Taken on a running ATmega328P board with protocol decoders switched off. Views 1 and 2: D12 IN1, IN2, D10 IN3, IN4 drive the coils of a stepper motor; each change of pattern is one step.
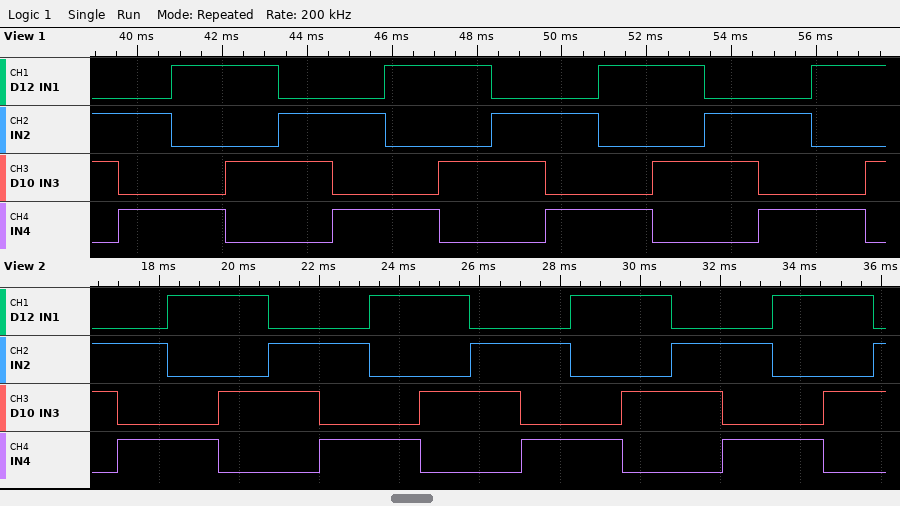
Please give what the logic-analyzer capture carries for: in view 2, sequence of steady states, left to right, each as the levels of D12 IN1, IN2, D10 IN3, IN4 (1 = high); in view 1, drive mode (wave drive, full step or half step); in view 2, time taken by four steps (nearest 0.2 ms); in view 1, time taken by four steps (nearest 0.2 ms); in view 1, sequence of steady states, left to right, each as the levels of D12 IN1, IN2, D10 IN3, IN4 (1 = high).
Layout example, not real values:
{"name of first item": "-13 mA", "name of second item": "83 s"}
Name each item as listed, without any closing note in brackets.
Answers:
{"in view 2, sequence of steady states, left to right, each as the levels of D12 IN1, IN2, D10 IN3, IN4": "0110 0101 1001 1010 0110 0101 1001 1010 0110 0101 1001 1010 0110 0101 1001 1010 0110", "in view 1, drive mode": "full step", "in view 2, time taken by four steps": "5.0 ms", "in view 1, time taken by four steps": "5.0 ms", "in view 1, sequence of steady states, left to right, each as the levels of D12 IN1, IN2, D10 IN3, IN4": "0110 0101 1001 1010 0110 0101 1001 1010 0110 0101 1001 1010 0110 0101 1001 1010"}
